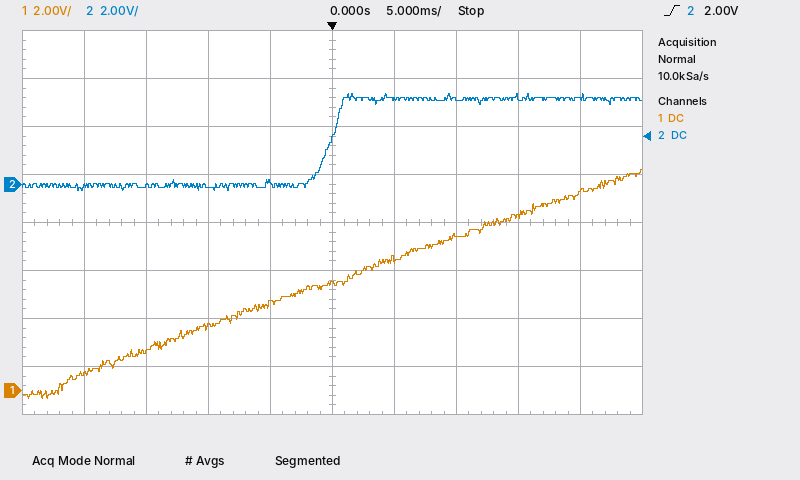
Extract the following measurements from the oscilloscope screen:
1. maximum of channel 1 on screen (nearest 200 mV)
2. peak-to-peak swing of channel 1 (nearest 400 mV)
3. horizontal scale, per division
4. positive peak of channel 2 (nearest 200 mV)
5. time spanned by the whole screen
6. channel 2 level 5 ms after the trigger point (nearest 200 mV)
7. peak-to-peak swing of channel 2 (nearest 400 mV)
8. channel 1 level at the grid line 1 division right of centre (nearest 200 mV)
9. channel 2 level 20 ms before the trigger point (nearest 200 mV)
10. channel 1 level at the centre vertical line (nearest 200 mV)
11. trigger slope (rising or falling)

9.2 V
9.6 V
5 ms
3.8 V
50 ms
3.6 V
4.0 V
5.4 V
-200 mV
4.4 V
rising
